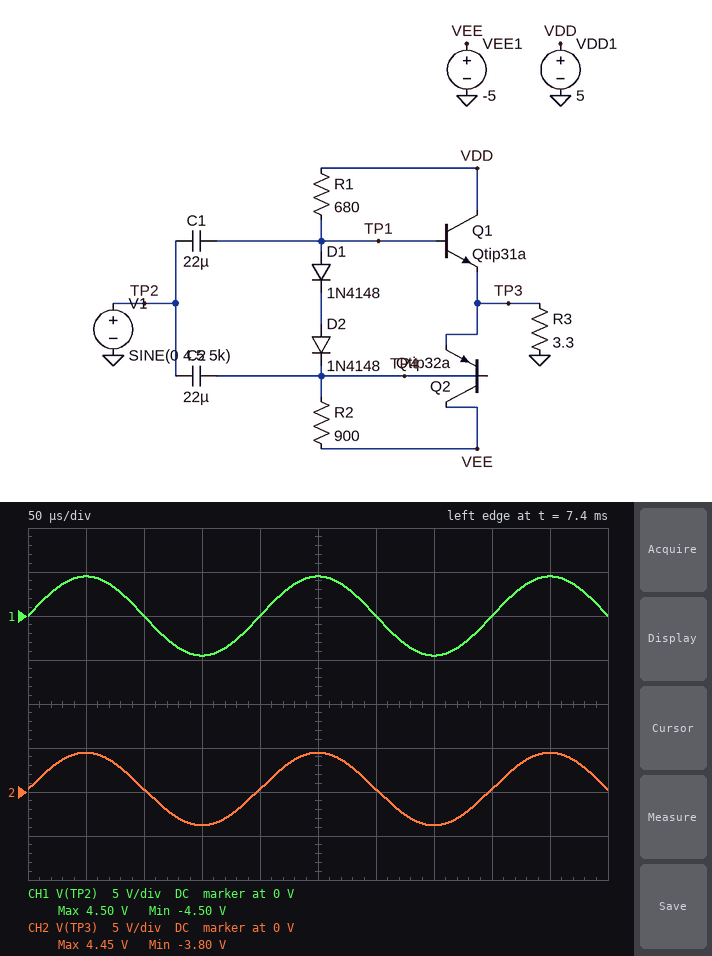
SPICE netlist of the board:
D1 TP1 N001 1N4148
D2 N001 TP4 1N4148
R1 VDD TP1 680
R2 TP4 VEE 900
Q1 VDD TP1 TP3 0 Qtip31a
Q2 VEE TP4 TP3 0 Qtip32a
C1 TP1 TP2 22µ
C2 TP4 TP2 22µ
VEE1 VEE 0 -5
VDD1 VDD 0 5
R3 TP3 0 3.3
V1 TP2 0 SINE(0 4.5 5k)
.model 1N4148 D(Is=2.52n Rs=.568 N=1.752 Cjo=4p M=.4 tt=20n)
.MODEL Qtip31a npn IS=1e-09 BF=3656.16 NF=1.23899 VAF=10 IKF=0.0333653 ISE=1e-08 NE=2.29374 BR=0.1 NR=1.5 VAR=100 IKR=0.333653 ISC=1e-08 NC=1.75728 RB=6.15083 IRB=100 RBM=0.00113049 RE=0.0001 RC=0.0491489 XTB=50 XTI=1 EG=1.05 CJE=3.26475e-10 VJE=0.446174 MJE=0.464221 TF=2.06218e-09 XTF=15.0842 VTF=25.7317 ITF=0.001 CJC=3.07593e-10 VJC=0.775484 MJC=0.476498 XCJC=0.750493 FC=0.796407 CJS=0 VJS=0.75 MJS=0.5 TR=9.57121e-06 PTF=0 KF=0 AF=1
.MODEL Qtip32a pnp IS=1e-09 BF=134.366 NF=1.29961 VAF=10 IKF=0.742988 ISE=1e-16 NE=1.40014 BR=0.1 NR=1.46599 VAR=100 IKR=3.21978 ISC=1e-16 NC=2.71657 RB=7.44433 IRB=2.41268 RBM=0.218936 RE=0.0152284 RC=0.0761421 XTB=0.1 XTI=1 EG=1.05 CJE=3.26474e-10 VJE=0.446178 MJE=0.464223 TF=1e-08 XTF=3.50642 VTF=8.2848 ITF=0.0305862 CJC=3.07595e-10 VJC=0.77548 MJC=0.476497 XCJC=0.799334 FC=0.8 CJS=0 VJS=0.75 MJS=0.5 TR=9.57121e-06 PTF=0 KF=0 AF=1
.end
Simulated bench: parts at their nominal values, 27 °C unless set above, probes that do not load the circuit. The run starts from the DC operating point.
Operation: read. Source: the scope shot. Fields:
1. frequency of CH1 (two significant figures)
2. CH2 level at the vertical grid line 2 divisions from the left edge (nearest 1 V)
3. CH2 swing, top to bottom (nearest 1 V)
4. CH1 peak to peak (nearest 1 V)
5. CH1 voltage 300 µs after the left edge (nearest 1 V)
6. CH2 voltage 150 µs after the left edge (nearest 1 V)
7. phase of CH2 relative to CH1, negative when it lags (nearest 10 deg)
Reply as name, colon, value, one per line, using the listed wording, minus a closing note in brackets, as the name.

frequency of CH1: 5.0 kHz
CH2 level at the vertical grid line 2 divisions from the left edge: 0 V
CH2 swing, top to bottom: 8 V
CH1 peak to peak: 9 V
CH1 voltage 300 µs after the left edge: 0 V
CH2 voltage 150 µs after the left edge: -4 V
phase of CH2 relative to CH1, negative when it lags: 0 deg
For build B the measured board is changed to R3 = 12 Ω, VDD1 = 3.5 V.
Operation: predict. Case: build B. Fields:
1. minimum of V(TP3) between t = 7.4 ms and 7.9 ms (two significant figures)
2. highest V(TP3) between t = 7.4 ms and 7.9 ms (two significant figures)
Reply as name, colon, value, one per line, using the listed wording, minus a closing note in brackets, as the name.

minimum of V(TP3) between t = 7.4 ms and 7.9 ms: -4.8 V
highest V(TP3) between t = 7.4 ms and 7.9 ms: 3.4 V
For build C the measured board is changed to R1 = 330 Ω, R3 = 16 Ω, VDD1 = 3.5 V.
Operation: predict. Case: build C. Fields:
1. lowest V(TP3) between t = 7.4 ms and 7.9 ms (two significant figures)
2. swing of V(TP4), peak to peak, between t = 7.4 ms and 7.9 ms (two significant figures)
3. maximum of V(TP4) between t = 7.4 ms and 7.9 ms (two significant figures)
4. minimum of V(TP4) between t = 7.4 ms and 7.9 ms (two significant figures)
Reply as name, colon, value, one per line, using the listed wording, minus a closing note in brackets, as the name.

lowest V(TP3) between t = 7.4 ms and 7.9 ms: -4.8 V
swing of V(TP4), peak to peak, between t = 7.4 ms and 7.9 ms: 9.0 V
maximum of V(TP4) between t = 7.4 ms and 7.9 ms: 3.4 V
minimum of V(TP4) between t = 7.4 ms and 7.9 ms: -5.6 V
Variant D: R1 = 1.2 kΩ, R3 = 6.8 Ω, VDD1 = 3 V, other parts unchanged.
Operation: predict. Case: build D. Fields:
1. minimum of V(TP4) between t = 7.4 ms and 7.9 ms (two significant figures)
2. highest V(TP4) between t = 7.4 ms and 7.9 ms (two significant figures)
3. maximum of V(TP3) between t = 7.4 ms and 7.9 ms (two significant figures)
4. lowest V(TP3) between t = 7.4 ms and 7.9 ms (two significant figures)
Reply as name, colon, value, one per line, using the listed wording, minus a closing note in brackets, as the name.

minimum of V(TP4) between t = 7.4 ms and 7.9 ms: -5.7 V
highest V(TP4) between t = 7.4 ms and 7.9 ms: 3.3 V
maximum of V(TP3) between t = 7.4 ms and 7.9 ms: 2.8 V
lowest V(TP3) between t = 7.4 ms and 7.9 ms: -4.8 V
